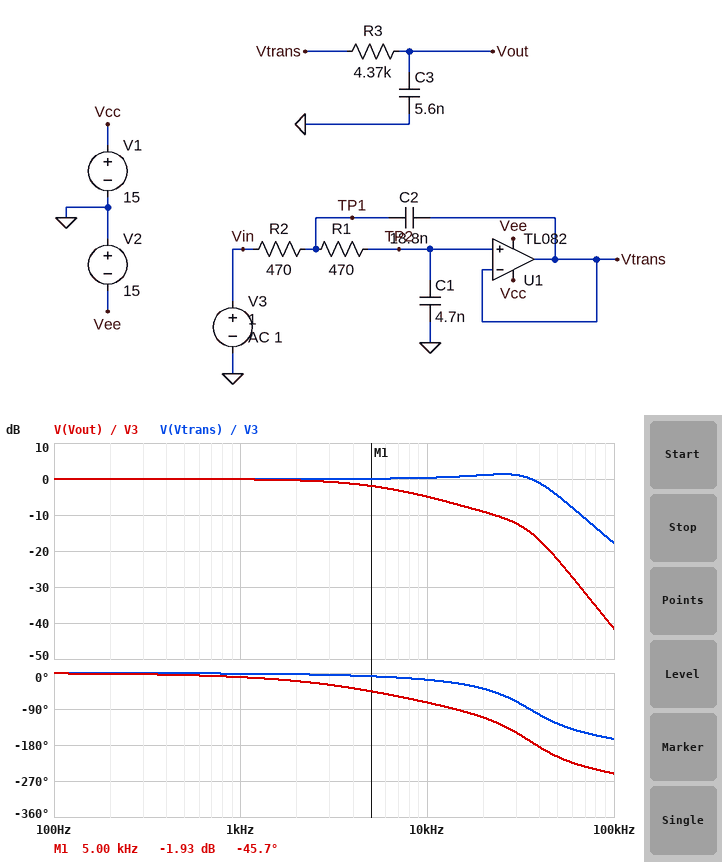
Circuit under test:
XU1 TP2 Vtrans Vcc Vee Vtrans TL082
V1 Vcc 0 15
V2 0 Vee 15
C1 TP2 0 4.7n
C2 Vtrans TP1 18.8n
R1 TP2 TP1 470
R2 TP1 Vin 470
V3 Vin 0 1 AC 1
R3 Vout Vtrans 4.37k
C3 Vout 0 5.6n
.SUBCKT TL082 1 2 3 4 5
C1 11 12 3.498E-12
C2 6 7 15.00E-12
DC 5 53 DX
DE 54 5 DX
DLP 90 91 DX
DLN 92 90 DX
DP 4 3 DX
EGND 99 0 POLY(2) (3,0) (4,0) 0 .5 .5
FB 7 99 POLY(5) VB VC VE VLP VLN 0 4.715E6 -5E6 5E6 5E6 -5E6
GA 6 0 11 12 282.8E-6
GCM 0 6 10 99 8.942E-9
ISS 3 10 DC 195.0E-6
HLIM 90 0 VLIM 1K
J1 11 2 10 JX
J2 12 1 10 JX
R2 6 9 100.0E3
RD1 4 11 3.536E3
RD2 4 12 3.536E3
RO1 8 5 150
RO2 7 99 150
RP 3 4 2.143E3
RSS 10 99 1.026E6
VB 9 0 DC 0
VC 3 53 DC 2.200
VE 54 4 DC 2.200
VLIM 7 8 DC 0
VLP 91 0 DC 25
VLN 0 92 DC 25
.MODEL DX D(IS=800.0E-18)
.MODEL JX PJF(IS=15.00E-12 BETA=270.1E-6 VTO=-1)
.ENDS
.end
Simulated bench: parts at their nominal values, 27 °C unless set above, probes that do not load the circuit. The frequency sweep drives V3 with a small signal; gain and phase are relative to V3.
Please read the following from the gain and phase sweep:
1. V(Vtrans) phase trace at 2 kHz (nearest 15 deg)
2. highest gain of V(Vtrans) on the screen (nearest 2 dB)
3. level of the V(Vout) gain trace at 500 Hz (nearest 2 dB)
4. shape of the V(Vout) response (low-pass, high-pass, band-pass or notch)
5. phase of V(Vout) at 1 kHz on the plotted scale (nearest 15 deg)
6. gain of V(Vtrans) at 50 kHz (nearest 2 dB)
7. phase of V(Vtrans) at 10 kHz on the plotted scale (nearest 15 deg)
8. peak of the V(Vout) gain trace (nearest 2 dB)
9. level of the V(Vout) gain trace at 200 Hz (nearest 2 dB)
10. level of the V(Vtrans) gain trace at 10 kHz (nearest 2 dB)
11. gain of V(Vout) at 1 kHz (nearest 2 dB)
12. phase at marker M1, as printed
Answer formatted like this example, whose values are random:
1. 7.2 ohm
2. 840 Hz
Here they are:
1. 0 deg
2. 2 dB
3. 0 dB
4. low-pass
5. -15 deg
6. -4 dB
7. -15 deg
8. 0 dB
9. 0 dB
10. 0 dB
11. 0 dB
12. -45.7 deg
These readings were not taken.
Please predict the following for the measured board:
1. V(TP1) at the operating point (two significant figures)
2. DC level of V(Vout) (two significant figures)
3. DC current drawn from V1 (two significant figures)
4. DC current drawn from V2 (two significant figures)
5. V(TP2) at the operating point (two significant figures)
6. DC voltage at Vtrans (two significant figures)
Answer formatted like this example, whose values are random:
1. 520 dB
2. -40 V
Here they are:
1. 1.0 V
2. 1.0 V
3. 14 mA
4. 14 mA
5. 1.0 V
6. 1.0 V
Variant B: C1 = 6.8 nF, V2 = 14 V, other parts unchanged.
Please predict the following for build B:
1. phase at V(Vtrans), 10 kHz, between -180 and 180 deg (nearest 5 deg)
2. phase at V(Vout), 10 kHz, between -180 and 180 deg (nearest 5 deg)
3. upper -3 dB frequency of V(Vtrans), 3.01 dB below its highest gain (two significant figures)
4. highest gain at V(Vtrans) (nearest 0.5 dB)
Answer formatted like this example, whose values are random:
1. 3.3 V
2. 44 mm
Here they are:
1. -25 deg
2. -80 deg
3. 33 kHz
4. 0.5 dB
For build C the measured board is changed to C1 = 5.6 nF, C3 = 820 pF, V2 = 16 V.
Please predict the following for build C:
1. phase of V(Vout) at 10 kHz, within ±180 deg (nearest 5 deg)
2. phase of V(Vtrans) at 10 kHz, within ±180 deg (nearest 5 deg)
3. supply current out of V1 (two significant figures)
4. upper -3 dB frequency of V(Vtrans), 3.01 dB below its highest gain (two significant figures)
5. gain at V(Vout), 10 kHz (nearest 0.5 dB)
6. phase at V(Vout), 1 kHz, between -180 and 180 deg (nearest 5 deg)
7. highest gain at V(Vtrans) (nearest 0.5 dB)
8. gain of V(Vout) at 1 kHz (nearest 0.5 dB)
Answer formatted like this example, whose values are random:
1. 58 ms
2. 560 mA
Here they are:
1. -35 deg
2. -20 deg
3. 15 mA
4. 38 kHz
5. 0 dB
6. -5 deg
7. 1.0 dB
8. 0 dB
